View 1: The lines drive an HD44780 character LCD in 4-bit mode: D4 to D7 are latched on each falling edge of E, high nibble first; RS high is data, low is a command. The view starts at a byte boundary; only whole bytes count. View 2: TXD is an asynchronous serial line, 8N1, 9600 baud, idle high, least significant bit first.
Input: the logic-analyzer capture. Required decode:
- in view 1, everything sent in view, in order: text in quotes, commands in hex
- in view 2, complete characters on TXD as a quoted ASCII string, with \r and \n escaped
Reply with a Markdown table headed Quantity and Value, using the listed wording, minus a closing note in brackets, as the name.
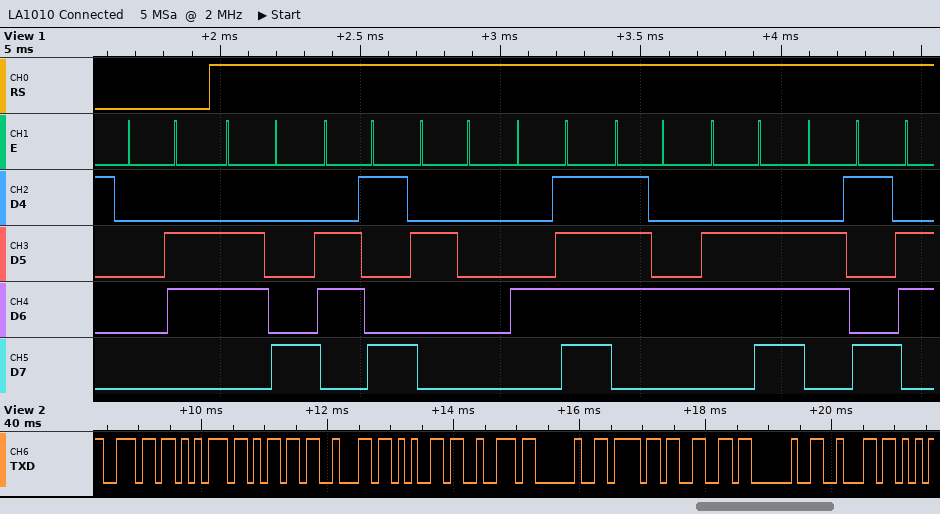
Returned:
| Quantity | Value |
|---|---|
| in view 1, everything sent in view, in order: text in quotes, commands in hex | 0x06 "hi Otni" |
| in view 2, complete characters on TXD as a quoted ASCII string, with \r and \n escaped | "number of b" |
